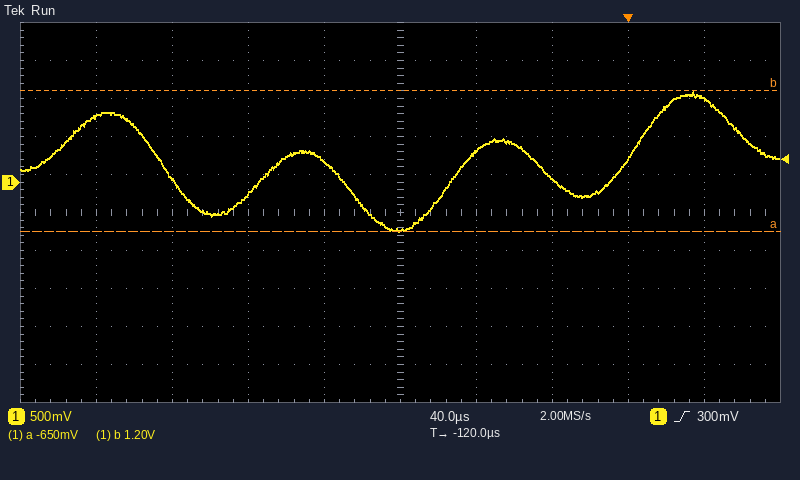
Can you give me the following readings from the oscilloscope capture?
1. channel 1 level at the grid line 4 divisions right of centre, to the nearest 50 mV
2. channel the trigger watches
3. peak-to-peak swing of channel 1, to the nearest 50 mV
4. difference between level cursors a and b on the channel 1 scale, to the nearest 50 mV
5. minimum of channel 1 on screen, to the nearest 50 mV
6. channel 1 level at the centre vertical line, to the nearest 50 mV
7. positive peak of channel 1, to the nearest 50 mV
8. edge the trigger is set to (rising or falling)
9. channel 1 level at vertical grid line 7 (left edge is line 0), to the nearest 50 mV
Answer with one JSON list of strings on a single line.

["1.10 V", "channel 1", "1.85 V", "1.85 V", "-650 mV", "-650 mV", "1.20 V", "rising", "50 mV"]
